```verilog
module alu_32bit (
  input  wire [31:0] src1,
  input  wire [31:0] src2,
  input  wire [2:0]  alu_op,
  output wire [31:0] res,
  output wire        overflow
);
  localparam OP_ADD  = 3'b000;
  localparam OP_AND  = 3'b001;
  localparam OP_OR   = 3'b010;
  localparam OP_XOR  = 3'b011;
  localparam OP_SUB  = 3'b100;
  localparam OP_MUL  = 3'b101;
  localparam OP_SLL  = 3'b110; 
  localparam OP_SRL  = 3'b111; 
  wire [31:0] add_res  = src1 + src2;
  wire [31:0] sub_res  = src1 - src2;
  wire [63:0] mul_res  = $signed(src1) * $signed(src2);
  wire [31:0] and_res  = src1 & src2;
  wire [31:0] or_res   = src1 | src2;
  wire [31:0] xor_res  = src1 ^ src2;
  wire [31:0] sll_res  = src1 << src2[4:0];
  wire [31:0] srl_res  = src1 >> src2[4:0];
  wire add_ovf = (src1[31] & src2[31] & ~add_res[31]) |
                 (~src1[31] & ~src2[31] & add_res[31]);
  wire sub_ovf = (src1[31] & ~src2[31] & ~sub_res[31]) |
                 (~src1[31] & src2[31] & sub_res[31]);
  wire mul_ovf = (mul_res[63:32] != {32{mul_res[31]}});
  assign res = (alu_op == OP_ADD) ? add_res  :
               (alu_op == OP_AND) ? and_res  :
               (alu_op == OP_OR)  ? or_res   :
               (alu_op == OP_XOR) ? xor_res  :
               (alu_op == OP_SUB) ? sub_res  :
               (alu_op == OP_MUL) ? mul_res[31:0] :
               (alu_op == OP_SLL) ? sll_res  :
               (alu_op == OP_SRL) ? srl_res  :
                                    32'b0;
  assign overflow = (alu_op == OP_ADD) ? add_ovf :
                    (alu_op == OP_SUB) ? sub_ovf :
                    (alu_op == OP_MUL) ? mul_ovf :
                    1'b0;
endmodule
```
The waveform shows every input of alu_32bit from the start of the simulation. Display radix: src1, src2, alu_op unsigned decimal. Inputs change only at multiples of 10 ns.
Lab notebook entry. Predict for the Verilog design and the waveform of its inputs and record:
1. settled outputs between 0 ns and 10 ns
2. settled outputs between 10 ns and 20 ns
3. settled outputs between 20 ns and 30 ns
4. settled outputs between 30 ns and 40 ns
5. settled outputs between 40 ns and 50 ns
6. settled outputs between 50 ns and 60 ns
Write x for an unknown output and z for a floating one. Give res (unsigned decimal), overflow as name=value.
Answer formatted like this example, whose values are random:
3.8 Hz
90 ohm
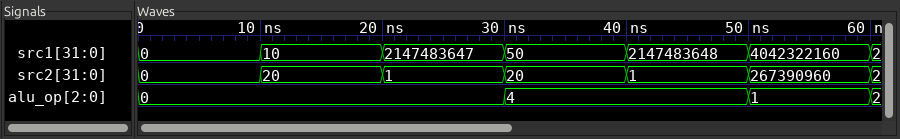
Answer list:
res=0, overflow=0
res=30, overflow=0
res=2147483648, overflow=1
res=30, overflow=0
res=2147483647, overflow=1
res=15728880, overflow=0
